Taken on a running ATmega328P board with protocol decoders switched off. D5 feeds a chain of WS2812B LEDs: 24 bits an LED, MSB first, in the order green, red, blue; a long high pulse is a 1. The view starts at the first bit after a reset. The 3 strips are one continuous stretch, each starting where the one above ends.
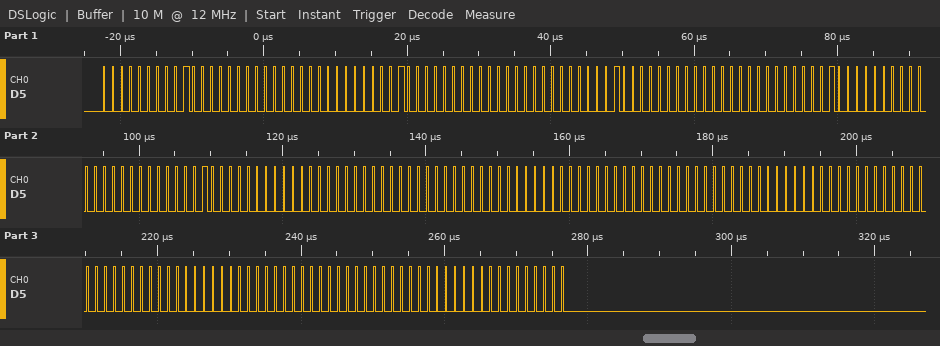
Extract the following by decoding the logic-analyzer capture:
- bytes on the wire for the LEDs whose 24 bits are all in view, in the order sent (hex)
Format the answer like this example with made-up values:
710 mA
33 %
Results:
00 40 00 00 40 00 00 40 00 00 40 00 00 40 00 00 00 00 00 00 00 00 00 00 00 00 00 00 00 00
